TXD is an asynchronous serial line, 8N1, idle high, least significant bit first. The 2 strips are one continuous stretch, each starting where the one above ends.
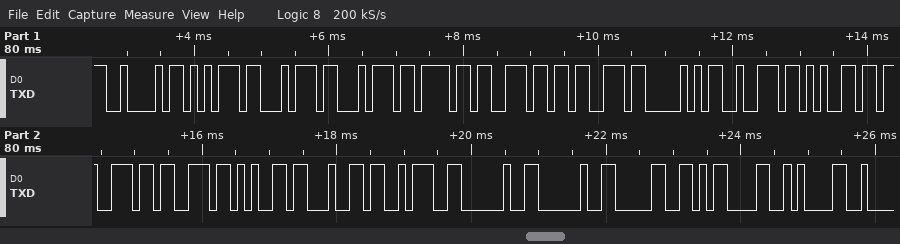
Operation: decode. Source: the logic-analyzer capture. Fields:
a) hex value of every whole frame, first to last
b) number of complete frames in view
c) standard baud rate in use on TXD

42 75 74 74 6F 6E 73 50 72 65 73 73 65 64 3A 20 20 30 0D 0A
20
9600 baud
